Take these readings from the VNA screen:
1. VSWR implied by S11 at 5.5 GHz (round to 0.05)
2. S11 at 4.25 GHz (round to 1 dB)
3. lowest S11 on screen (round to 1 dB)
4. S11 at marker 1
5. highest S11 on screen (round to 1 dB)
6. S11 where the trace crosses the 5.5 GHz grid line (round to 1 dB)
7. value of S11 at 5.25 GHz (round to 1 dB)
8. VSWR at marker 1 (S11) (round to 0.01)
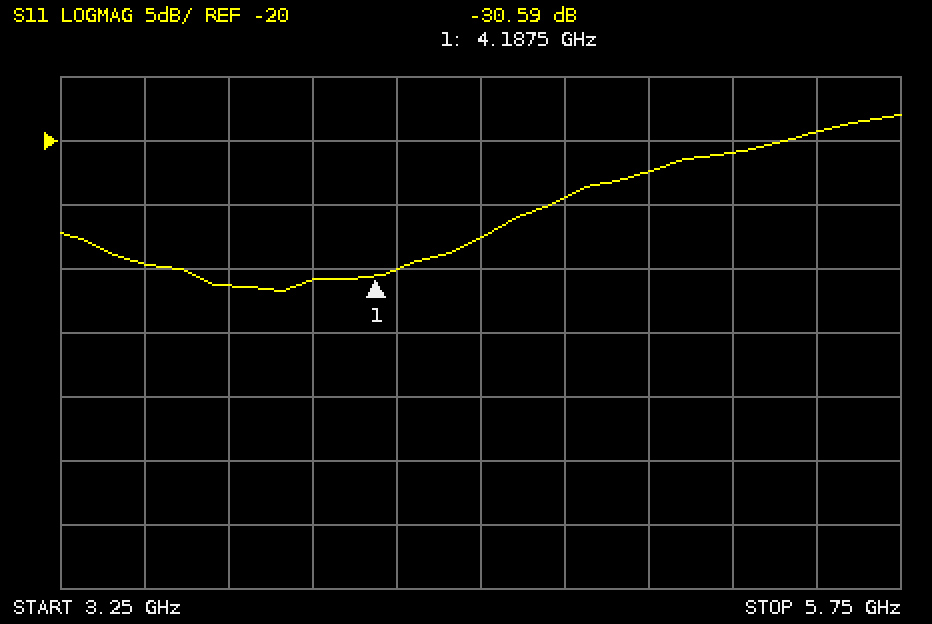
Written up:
1.25
-30 dB
-32 dB
-30.59 dB
-18 dB
-19 dB
-21 dB
1.06
